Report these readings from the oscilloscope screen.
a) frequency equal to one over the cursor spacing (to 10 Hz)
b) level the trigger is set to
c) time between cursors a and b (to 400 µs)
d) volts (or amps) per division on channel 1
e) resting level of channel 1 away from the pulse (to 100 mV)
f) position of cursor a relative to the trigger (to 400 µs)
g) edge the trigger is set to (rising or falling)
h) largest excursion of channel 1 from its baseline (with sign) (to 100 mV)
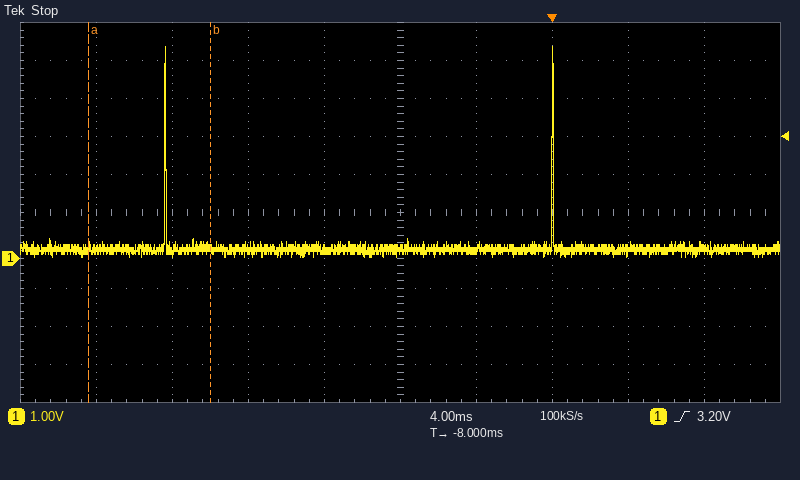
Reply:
160 Hz
3.20 V
6.4 ms
1 V
200 mV
-24.4 ms
rising
+5.3 V
